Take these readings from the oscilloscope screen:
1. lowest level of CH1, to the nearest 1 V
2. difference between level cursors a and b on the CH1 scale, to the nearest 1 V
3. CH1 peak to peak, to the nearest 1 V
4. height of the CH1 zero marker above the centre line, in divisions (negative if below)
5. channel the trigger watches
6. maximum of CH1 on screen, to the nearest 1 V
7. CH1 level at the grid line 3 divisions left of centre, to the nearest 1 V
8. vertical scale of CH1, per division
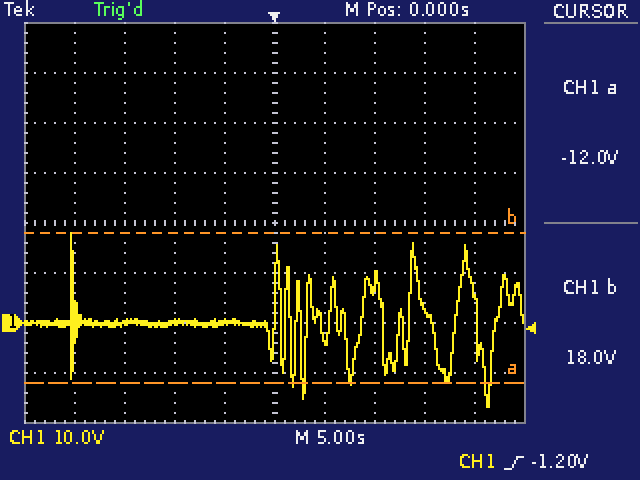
-17 V
30 V
35 V
-2.0 div
CH1
18 V
0 V
10 V
